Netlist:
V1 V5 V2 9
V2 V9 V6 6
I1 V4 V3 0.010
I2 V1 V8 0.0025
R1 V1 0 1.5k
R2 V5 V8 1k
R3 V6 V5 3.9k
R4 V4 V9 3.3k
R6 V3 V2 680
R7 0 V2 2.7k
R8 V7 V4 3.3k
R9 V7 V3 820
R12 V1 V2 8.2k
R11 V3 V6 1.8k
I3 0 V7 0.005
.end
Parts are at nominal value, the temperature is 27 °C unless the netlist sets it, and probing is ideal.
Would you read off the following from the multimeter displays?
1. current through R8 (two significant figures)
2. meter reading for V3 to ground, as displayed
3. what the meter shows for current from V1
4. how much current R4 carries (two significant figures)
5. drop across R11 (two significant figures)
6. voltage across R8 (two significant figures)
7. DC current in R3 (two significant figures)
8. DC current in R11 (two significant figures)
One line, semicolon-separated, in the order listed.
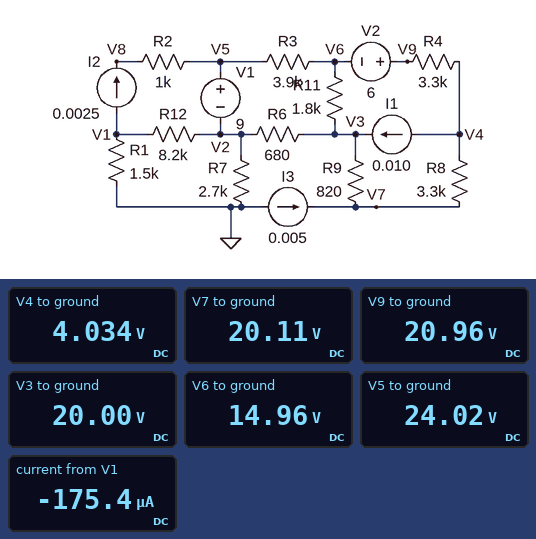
4.9 mA; 20.00 V; -175.4 µA; 5.1 mA; 5.0 V; 16 V; 2.3 mA; 2.8 mA
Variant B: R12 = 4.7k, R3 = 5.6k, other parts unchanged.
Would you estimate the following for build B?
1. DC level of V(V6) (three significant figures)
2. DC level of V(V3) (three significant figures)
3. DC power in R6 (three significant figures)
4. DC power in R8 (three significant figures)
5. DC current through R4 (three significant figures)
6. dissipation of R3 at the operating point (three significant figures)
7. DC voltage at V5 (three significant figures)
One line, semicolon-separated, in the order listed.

11.8 V; 17.6 V; 31.6 mW; 81.6 mW; 5.03 mA; 18.4 mW; 22.0 V
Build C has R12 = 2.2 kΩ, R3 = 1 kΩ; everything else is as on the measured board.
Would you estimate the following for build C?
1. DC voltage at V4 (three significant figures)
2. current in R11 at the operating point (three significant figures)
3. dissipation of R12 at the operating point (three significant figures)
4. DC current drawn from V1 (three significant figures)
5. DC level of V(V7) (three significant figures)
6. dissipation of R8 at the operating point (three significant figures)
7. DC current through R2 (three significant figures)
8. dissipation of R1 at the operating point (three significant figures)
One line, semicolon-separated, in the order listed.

2.33 V; 1.07 mA; 30.9 mW; 1.98 mA; 17.0 V; 65.4 mW; 2.50 mA; 2.34 mW
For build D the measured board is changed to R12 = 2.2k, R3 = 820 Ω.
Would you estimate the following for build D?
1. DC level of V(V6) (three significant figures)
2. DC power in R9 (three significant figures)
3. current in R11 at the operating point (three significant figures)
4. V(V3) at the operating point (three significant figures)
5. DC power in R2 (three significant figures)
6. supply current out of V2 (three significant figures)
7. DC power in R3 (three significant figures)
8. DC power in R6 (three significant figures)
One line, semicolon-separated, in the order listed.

15.2 V; 298 µW; 850 µA; 16.8 V; 6.25 mW; 5.60 mA; 18.5 mW; 64.7 mW
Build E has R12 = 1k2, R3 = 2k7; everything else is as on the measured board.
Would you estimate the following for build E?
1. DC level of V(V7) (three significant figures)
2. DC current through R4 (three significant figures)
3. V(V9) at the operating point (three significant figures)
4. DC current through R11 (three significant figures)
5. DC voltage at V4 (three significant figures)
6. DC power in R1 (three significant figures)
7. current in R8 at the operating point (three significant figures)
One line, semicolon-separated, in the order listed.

13.8 V; 5.24 mA; 15.4 V; 2.34 mA; -1.88 V; 5.67 mW; 4.76 mA
